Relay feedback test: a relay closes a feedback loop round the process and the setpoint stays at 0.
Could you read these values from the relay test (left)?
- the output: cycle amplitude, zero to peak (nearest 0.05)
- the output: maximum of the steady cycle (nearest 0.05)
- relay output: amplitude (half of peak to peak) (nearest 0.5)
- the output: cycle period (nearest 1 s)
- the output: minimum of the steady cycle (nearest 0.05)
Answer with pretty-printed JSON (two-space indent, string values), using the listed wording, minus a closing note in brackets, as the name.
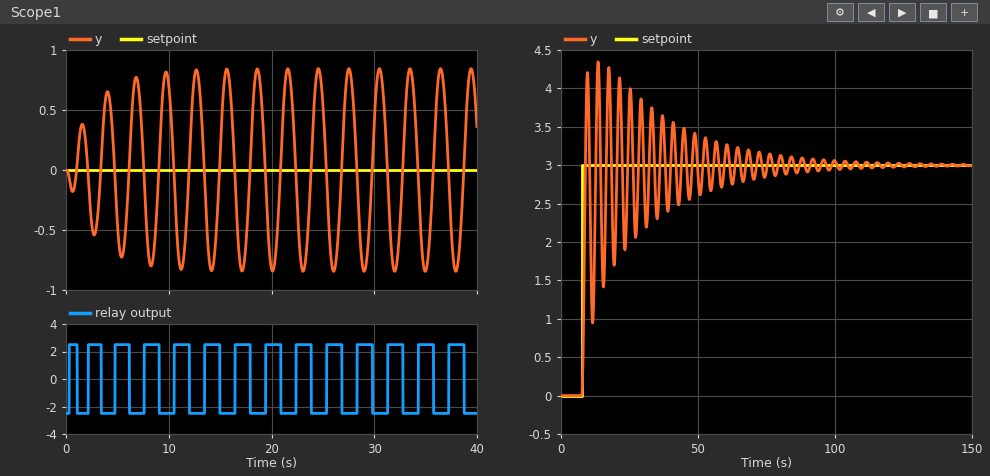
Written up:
{
  "the output: cycle amplitude, zero to peak": "0.85",
  "the output: maximum of the steady cycle": "0.85",
  "relay output: amplitude (half of peak to peak)": "2.5",
  "the output: cycle period": "3 s",
  "the output: minimum of the steady cycle": "-0.85"
}
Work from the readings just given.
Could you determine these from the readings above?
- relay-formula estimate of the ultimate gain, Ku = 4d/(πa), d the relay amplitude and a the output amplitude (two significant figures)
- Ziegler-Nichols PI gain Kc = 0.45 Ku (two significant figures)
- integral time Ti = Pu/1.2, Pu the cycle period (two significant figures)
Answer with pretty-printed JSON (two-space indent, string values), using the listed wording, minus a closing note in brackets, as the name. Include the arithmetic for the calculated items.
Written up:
{
  "relay-formula estimate of the ultimate gain, Ku = 4d/(πa), d the relay amplitude and a the output amplitude": "4 × 2.5 / (π × 0.85) = 3.7",
  "Ziegler-Nichols PI gain Kc = 0.45 Ku": "0.45 × 3.7 = 1.7",
  "integral time Ti = Pu/1.2, Pu the cycle period": "3 / 1.2 = 2.5 s"
}
